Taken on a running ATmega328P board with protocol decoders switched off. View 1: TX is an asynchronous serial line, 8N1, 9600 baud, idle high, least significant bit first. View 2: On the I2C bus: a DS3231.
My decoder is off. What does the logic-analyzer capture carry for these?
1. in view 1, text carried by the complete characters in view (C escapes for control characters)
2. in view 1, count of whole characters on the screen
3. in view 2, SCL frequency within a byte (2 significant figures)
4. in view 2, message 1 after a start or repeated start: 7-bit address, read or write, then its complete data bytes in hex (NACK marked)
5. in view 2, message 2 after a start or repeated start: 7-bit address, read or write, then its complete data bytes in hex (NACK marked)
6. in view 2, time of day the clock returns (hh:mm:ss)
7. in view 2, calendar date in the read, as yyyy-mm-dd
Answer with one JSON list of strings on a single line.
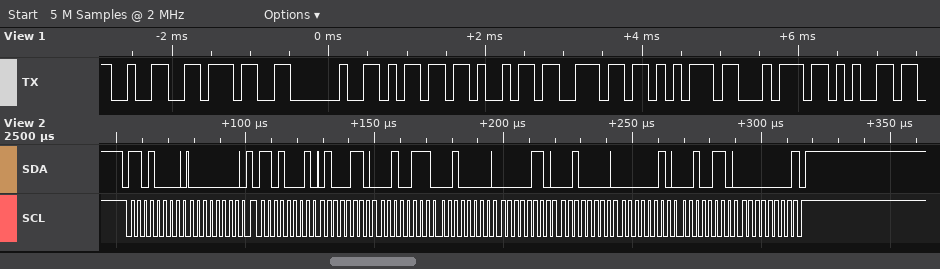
["\"27 minute\"", "9", "400 kHz", "0x68 write: 00", "0x68 read: 46 27 20 06 20 02 26 00 NACK", "20:27:46", "2026-02-20"]
